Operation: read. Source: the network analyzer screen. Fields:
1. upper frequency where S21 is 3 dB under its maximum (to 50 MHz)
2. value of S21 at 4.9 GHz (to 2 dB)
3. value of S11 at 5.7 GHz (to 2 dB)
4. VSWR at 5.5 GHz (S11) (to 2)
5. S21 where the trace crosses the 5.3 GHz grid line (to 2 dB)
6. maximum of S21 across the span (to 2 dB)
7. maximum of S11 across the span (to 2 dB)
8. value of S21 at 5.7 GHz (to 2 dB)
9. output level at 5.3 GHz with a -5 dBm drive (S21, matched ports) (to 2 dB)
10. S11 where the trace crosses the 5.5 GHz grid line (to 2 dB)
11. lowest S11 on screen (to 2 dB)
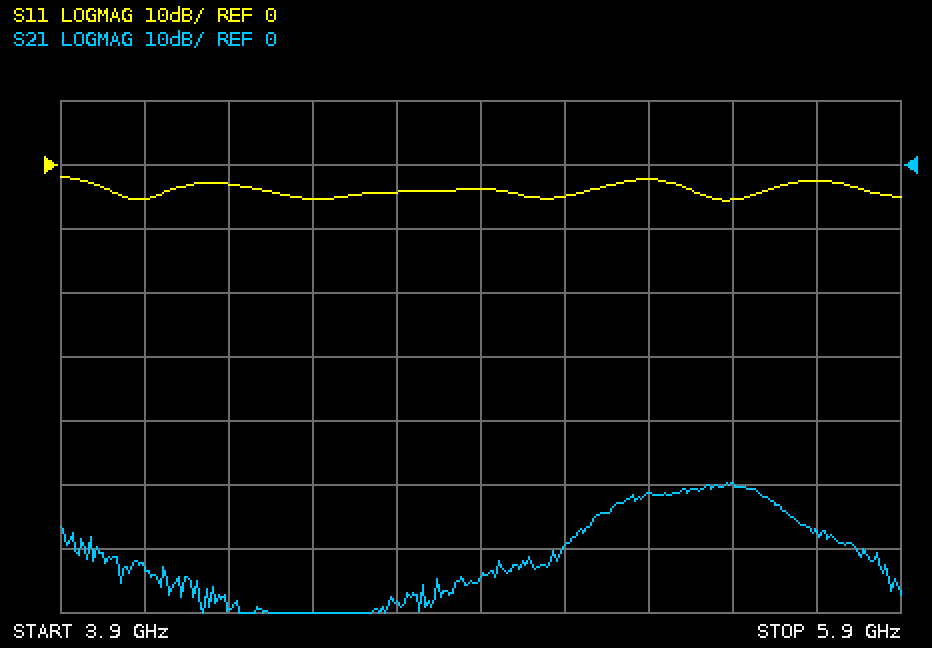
5.60 GHz
-64 dB
-2 dB
4
-52 dB
-50 dB
-2 dB
-58 dB
-56 dBm
-6 dB
-6 dB
